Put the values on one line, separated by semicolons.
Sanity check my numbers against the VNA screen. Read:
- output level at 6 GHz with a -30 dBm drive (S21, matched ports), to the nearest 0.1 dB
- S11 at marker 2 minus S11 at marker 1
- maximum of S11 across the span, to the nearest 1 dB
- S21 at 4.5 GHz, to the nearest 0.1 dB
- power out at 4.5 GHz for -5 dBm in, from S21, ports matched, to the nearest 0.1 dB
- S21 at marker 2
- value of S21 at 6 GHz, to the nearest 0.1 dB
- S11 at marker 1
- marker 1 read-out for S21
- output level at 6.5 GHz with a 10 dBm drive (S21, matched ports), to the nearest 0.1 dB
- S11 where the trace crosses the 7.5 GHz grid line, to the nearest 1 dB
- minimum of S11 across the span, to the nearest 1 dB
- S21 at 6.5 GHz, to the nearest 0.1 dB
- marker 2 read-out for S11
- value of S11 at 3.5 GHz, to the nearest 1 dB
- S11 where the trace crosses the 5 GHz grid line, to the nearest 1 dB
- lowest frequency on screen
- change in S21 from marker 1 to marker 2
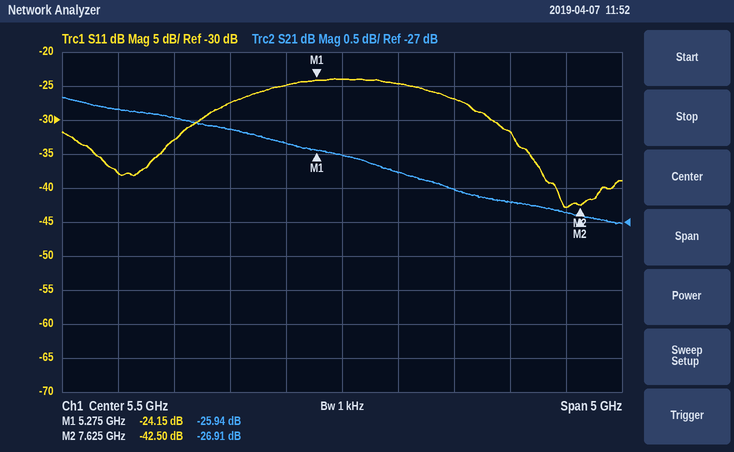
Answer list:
-56.3 dBm; -18.35 dB; -24 dB; -25.6 dB; -30.6 dBm; -26.91 dB; -26.3 dB; -24.15 dB; -25.94 dB; -16.5 dBm; -43 dB; -43 dB; -26.5 dB; -42.50 dB; -38 dB; -25 dB; 3 GHz; -0.97 dB
